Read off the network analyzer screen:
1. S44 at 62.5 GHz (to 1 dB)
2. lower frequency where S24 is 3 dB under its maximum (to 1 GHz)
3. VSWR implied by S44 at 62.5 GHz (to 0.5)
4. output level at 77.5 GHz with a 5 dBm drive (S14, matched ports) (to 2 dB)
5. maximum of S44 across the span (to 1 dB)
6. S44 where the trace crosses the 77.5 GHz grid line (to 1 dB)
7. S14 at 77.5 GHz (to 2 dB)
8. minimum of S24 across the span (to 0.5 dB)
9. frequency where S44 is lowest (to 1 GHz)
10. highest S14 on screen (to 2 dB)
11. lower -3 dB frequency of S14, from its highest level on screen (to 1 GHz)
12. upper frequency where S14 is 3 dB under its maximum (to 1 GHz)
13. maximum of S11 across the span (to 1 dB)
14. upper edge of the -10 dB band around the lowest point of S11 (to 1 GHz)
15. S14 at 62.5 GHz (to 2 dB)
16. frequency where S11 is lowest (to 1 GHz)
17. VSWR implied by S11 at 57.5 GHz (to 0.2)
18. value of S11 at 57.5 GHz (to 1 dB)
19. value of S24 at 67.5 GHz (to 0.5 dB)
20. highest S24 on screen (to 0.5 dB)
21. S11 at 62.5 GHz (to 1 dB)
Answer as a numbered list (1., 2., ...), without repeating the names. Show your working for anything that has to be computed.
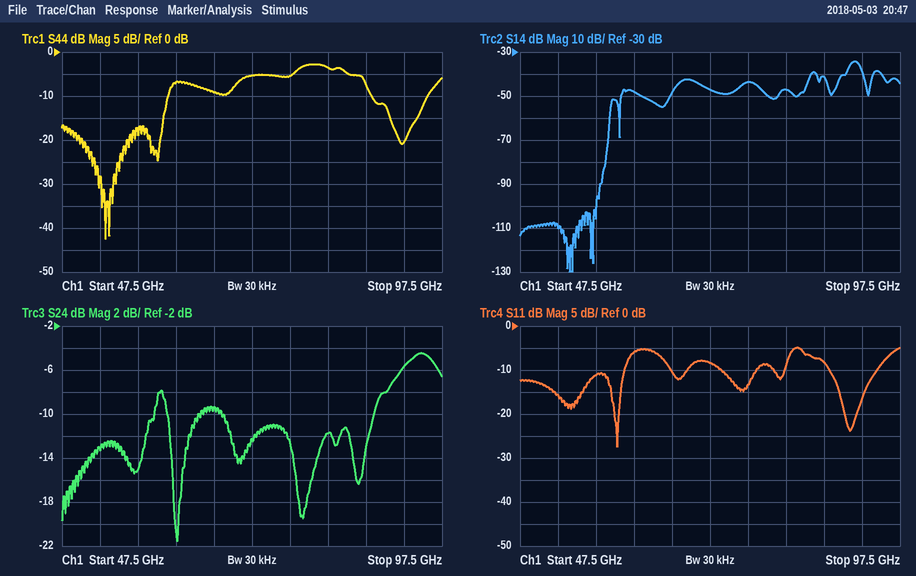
1. -7 dB
2. 91 GHz
3. |Γ| = 10^(-7/20) = 0.4467; VSWR = (1 + 0.4467)/(1 − 0.4467) ≈ 2.61, so 2.5 to the nearest 0.5
4. 5 dBm + (-44 dB) = -38 dBm
5. -3 dB
6. -5 dB
7. -44 dB
8. -21.5 dB
9. 53 GHz
10. -34 dB
11. 91 GHz
12. 92 GHz
13. -5 dB
14. 61 GHz
15. -48 dB
16. 60 GHz
17. |Γ| = 10^(-11/20) = 0.2818; VSWR = (1 + 0.2818)/(1 − 0.2818) ≈ 1.8
18. -11 dB
19. -9.5 dB
20. -4.5 dB
21. -6 dB
